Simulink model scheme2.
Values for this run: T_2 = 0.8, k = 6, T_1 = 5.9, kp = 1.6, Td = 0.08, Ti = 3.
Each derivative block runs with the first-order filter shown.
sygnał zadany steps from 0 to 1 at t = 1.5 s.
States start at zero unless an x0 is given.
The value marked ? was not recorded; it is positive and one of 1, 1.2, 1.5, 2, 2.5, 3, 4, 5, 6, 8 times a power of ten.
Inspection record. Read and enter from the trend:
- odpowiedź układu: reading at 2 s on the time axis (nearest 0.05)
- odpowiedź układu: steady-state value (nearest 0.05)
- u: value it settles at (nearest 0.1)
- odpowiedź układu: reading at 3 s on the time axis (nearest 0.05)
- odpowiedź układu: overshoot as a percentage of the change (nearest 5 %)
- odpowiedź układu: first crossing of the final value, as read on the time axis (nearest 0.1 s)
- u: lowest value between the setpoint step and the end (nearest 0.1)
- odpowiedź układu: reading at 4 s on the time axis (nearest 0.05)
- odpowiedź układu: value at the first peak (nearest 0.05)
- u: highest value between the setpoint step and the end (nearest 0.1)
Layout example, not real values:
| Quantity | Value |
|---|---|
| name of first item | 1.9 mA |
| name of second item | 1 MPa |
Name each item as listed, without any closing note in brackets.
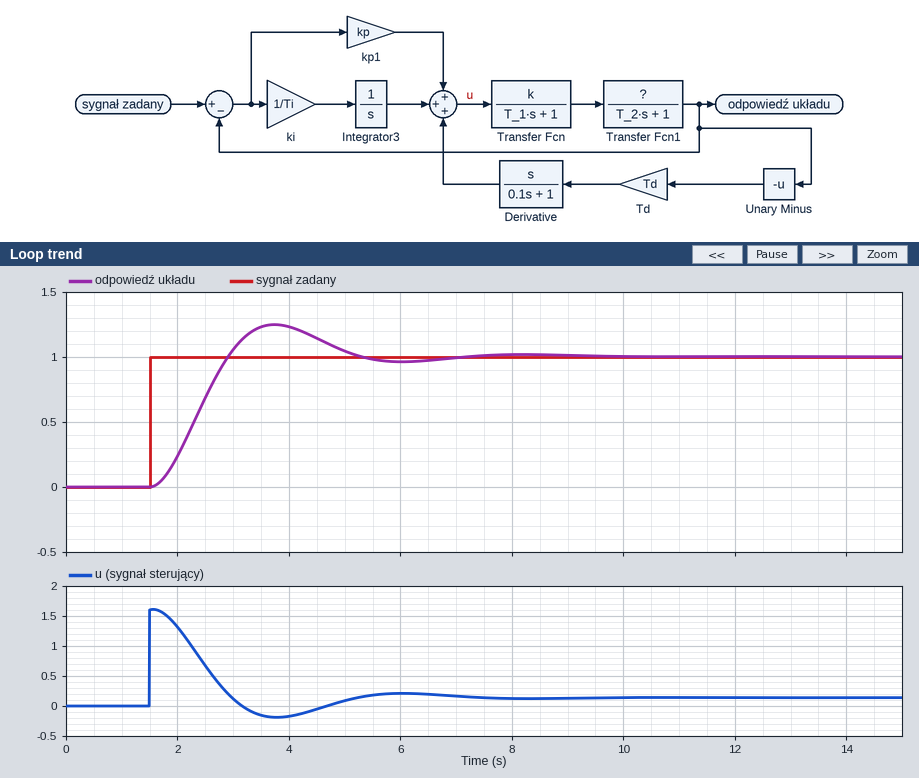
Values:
| Quantity | Value |
|---|---|
| odpowiedź układu: reading at 2 s on the time axis | 0.25 |
| odpowiedź układu: steady-state value | 1.00 |
| u: value it settles at | 0.1 |
| odpowiedź układu: reading at 3 s on the time axis | 1.05 |
| odpowiedź układu: overshoot as a percentage of the change | 25 % |
| odpowiedź układu: first crossing of the final value, as read on the time axis | 2.9 s |
| u: lowest value between the setpoint step and the end | -0.2 |
| odpowiedź układu: reading at 4 s on the time axis | 1.25 |
| odpowiedź układu: value at the first peak | 1.25 |
| u: highest value between the setpoint step and the end | 1.6 |
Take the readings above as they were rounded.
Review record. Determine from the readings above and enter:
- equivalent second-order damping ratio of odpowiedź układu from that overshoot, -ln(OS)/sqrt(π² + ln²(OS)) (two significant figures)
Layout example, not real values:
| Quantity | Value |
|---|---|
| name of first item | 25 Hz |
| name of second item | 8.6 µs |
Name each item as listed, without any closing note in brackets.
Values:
| Quantity | Value |
|---|---|
| equivalent second-order damping ratio of odpowiedź układu from that overshoot, -ln(OS)/sqrt(π² + ln²(OS)) | 0.40 |
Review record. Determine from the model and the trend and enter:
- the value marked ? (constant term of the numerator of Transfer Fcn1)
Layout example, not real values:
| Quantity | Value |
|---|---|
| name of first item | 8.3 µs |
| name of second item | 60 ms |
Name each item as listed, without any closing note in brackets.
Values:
| Quantity | Value |
|---|---|
| the value marked ? | 1.2 |
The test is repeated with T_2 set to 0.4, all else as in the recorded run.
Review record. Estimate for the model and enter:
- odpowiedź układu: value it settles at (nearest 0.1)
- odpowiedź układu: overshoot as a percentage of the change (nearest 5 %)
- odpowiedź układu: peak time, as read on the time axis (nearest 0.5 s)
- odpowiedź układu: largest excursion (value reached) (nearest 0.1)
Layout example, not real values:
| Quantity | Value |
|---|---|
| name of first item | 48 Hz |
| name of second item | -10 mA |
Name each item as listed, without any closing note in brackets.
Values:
| Quantity | Value |
|---|---|
| odpowiedź układu: value it settles at | 1.0 |
| odpowiedź układu: overshoot as a percentage of the change | 10 % |
| odpowiedź układu: peak time, as read on the time axis | 3.5 s |
| odpowiedź układu: largest excursion (value reached) | 1.1 |
